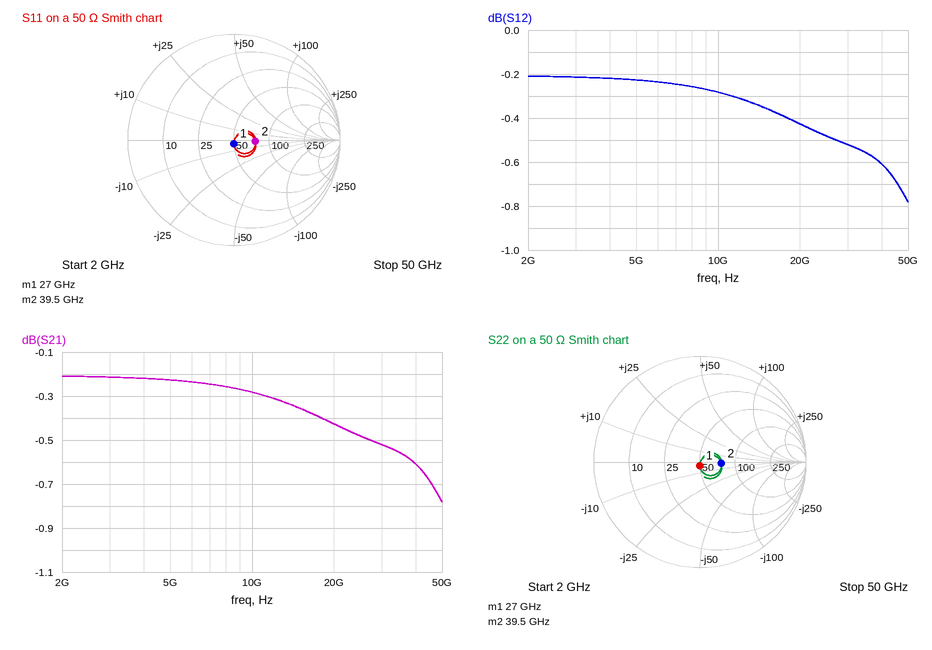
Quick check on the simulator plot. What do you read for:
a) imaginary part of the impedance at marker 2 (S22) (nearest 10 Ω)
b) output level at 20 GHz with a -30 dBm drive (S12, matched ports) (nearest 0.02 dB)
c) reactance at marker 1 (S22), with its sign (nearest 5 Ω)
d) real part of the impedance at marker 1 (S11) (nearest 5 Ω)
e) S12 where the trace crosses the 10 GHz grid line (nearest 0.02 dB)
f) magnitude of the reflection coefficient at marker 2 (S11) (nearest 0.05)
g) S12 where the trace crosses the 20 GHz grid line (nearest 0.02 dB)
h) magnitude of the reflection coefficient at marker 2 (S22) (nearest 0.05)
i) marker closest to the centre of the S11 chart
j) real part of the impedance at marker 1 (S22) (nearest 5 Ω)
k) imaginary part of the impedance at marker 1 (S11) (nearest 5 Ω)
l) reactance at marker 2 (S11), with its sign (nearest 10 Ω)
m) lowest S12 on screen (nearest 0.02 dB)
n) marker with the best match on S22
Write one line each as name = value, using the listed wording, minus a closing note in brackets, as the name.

imaginary part of the impedance at marker 2 (S22) = 0 Ω
output level at 20 GHz with a -30 dBm drive (S12, matched ports) = -30.42 dBm
reactance at marker 1 (S22), with its sign = -5 Ω
real part of the impedance at marker 1 (S11) = 50 Ω
S12 where the trace crosses the 10 GHz grid line = -0.28 dB
magnitude of the reflection coefficient at marker 2 (S11) = 0.20
S12 where the trace crosses the 20 GHz grid line = -0.42 dB
magnitude of the reflection coefficient at marker 2 (S22) = 0.20
marker closest to the centre of the S11 chart = marker 1
real part of the impedance at marker 1 (S22) = 50 Ω
imaginary part of the impedance at marker 1 (S11) = -5 Ω
reactance at marker 2 (S11), with its sign = 0 Ω
lowest S12 on screen = -0.78 dB
marker with the best match on S22 = marker 1
